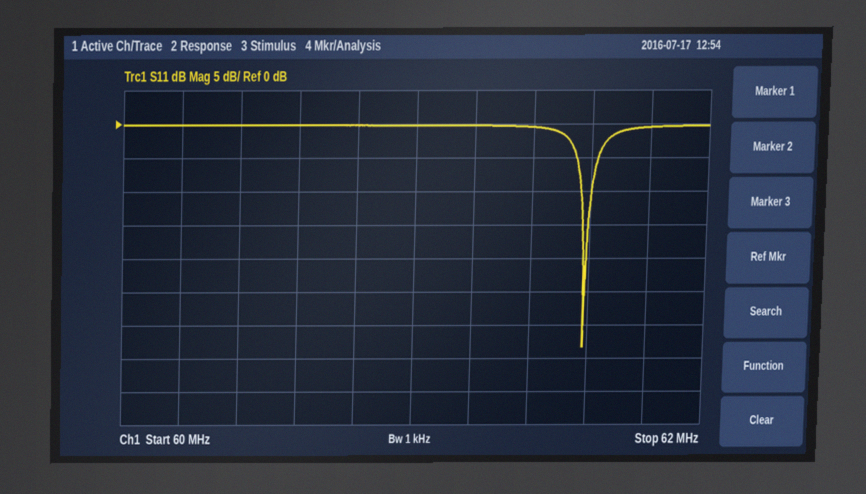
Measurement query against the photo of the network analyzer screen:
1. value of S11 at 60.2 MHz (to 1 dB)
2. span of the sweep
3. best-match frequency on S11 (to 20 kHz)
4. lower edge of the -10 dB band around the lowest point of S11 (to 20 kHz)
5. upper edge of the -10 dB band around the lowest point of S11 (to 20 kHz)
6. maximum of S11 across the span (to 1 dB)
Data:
0 dB
2 MHz
61.58 MHz
61.56 MHz
61.60 MHz
0 dB
